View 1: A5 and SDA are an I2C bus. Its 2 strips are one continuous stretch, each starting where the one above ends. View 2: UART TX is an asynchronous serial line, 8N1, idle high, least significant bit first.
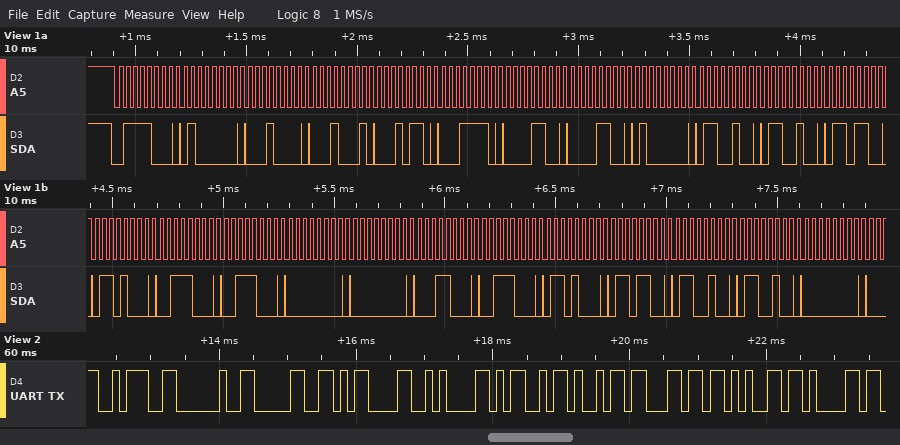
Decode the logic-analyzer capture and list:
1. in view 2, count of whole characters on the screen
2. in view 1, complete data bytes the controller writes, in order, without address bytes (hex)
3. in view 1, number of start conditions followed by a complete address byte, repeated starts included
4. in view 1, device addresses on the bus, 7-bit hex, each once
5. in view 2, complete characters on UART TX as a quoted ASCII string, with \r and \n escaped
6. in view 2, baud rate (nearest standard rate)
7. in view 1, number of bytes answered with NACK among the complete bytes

10
40 10 11 16 1E 0C 0C 40 64 64 6C 68 38 38 00 00 18 38 68 6C 64 64 00
1
0x3C
": 0\r\nMilea"
9600 baud
0
